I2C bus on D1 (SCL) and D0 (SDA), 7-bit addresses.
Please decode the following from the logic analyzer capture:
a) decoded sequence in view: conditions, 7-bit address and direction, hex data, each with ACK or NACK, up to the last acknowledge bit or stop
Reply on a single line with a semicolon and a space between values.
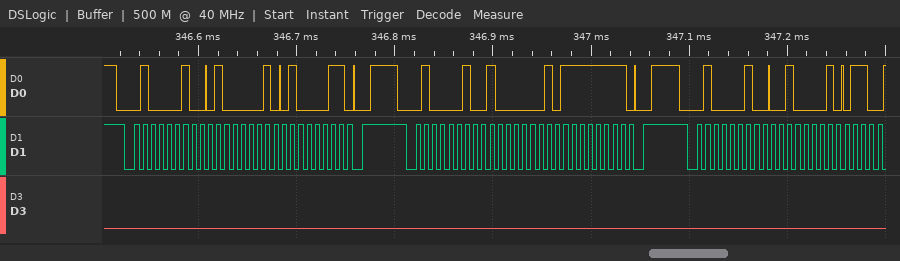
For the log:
start, address 21 write ACK, 41 ACK, 43 ACK, stop, start, address 21 write ACK, 81 ACK, FF ACK, stop, start, address 21 write ACK, 21 ACK
